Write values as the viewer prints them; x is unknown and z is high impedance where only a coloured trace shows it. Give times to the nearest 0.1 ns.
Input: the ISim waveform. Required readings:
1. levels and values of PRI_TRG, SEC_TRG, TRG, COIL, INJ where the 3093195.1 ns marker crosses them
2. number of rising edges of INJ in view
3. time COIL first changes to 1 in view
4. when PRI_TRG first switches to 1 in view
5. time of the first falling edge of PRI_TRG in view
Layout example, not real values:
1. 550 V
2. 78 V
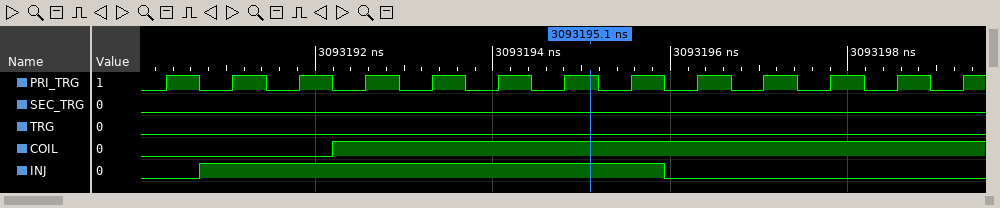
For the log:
1. PRI_TRG=1, SEC_TRG=0, TRG=0, COIL=1, INJ=1
2. 1
3. 3093192.2 ns
4. 3093190.3 ns
5. 3093190.7 ns
